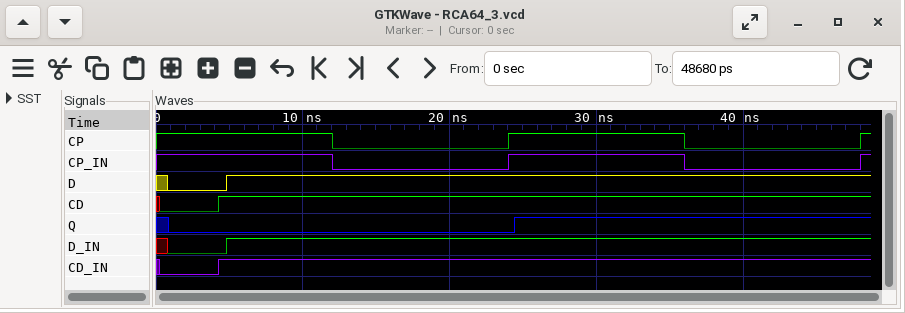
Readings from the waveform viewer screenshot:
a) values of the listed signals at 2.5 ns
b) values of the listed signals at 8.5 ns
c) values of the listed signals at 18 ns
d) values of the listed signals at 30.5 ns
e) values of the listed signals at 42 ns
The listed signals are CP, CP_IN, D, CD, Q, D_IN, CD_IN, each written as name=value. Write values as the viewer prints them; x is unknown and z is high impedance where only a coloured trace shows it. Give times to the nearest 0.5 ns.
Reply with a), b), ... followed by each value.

a) CP=1, CP_IN=1, D=0, CD=0, Q=0, D_IN=0, CD_IN=0
b) CP=1, CP_IN=1, D=1, CD=1, Q=0, D_IN=1, CD_IN=1
c) CP=0, CP_IN=0, D=1, CD=1, Q=0, D_IN=1, CD_IN=1
d) CP=1, CP_IN=1, D=1, CD=1, Q=1, D_IN=1, CD_IN=1
e) CP=0, CP_IN=0, D=1, CD=1, Q=1, D_IN=1, CD_IN=1
